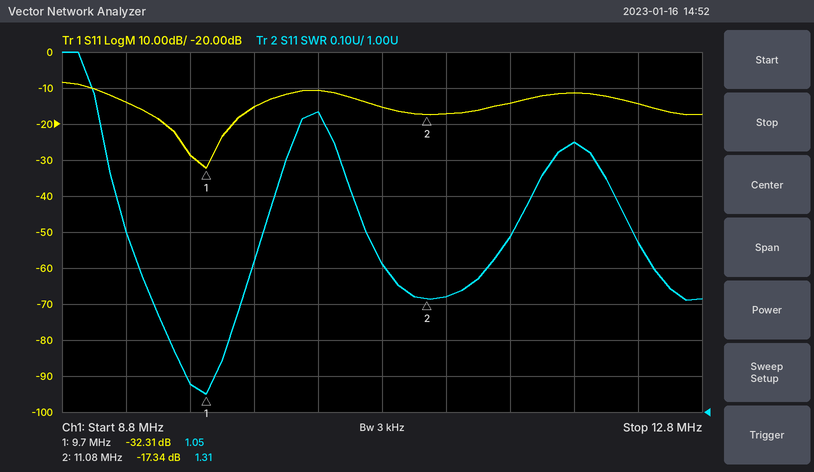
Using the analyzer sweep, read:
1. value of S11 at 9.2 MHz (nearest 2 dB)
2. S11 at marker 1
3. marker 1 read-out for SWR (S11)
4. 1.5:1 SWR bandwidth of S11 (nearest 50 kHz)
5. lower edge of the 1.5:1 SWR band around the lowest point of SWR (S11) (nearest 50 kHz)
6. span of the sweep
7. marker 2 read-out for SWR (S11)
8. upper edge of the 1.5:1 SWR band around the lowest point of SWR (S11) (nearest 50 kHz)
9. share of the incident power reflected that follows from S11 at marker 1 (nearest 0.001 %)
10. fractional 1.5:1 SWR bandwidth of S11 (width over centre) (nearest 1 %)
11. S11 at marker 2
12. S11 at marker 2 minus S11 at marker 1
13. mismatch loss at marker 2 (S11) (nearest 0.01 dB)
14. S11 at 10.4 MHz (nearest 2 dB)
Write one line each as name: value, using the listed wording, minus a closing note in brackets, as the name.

value of S11 at 9.2 MHz: -14 dB
S11 at marker 1: -32.31 dB
marker 1 read-out for SWR: 1.05
1.5:1 SWR bandwidth of S11: 850 kHz
lower edge of the 1.5:1 SWR band around the lowest point of SWR (S11): 9.20 MHz
span of the sweep: 4 MHz
marker 2 read-out for SWR: 1.31
upper edge of the 1.5:1 SWR band around the lowest point of SWR (S11): 10.05 MHz
share of the incident power reflected that follows from S11 at marker 1: 0.059 %
fractional 1.5:1 SWR bandwidth of S11 (width over centre): 9 %
S11 at marker 2: -17.34 dB
S11 at marker 2 minus S11 at marker 1: 14.97 dB
mismatch loss at marker 2 (S11): 0.08 dB
S11 at 10.4 MHz: -10 dB
